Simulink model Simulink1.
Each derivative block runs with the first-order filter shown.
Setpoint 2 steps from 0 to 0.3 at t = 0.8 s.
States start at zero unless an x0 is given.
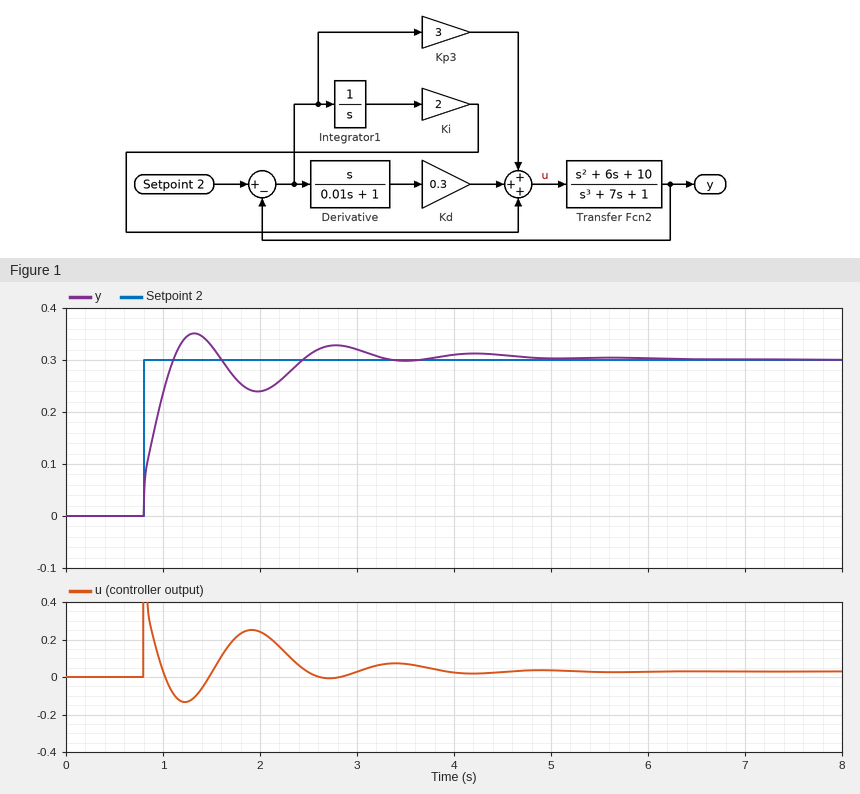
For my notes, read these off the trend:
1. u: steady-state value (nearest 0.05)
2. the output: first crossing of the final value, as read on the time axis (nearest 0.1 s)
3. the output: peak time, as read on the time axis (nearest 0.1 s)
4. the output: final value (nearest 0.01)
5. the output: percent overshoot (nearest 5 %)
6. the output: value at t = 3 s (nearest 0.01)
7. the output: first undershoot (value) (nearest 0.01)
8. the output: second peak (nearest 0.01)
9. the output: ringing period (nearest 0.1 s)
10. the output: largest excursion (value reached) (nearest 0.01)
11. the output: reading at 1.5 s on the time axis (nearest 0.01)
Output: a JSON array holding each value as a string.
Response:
["0.05", "1.1 s", "1.3 s", "0.30", "15 %", "0.32", "0.24", "0.33", "1.5 s", "0.35", "0.33"]
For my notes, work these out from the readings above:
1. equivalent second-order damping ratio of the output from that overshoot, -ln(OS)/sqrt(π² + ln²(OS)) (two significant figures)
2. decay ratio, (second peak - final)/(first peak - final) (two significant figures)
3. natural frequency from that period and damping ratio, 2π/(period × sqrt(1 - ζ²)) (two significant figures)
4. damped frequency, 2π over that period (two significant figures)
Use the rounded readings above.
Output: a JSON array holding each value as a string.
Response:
["0.52", "0.60", "4.9 rad/s", "4.2 rad/s"]
